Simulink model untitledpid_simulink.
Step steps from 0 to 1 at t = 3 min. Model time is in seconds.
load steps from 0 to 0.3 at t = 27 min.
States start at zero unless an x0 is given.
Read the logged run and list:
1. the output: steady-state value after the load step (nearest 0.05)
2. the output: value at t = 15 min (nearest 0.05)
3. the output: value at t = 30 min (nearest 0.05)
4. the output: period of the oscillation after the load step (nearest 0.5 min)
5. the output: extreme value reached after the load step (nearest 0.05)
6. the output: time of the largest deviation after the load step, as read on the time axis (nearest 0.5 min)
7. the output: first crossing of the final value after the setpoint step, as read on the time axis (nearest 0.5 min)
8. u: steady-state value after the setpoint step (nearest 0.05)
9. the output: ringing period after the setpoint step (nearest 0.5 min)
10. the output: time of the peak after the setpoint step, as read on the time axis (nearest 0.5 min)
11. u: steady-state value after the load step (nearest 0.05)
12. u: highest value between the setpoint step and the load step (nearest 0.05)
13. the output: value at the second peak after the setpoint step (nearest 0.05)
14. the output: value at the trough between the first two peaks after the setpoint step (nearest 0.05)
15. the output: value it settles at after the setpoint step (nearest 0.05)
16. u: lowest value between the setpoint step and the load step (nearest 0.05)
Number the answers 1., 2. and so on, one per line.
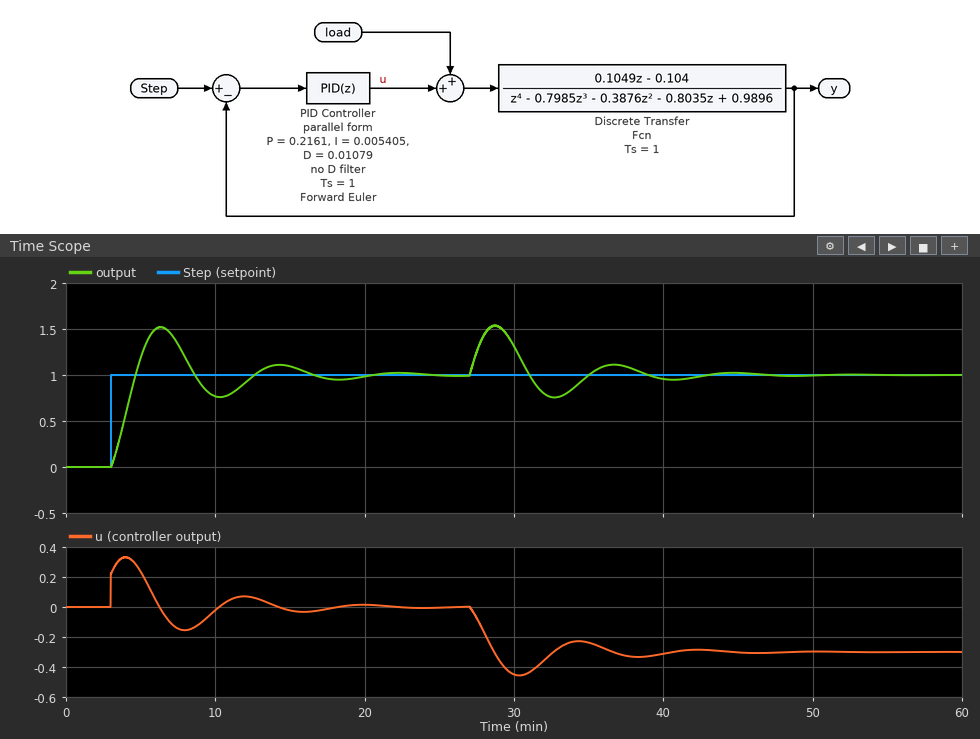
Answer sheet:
1. 1.00
2. 1.10
3. 1.30
4. 8.0 min
5. 1.55
6. 28.5 min
7. 4.5 min
8. 0.00
9. 8.0 min
10. 6.5 min
11. -0.30
12. 0.35
13. 1.10
14. 0.75
15. 1.00
16. -0.15
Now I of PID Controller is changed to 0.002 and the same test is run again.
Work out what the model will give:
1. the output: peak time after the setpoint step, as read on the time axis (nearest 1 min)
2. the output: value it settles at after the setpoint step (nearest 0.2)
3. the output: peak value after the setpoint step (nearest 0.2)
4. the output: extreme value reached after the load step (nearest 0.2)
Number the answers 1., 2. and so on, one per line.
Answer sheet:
1. 8 min
2. 1.0
3. 1.4
4. 1.8
